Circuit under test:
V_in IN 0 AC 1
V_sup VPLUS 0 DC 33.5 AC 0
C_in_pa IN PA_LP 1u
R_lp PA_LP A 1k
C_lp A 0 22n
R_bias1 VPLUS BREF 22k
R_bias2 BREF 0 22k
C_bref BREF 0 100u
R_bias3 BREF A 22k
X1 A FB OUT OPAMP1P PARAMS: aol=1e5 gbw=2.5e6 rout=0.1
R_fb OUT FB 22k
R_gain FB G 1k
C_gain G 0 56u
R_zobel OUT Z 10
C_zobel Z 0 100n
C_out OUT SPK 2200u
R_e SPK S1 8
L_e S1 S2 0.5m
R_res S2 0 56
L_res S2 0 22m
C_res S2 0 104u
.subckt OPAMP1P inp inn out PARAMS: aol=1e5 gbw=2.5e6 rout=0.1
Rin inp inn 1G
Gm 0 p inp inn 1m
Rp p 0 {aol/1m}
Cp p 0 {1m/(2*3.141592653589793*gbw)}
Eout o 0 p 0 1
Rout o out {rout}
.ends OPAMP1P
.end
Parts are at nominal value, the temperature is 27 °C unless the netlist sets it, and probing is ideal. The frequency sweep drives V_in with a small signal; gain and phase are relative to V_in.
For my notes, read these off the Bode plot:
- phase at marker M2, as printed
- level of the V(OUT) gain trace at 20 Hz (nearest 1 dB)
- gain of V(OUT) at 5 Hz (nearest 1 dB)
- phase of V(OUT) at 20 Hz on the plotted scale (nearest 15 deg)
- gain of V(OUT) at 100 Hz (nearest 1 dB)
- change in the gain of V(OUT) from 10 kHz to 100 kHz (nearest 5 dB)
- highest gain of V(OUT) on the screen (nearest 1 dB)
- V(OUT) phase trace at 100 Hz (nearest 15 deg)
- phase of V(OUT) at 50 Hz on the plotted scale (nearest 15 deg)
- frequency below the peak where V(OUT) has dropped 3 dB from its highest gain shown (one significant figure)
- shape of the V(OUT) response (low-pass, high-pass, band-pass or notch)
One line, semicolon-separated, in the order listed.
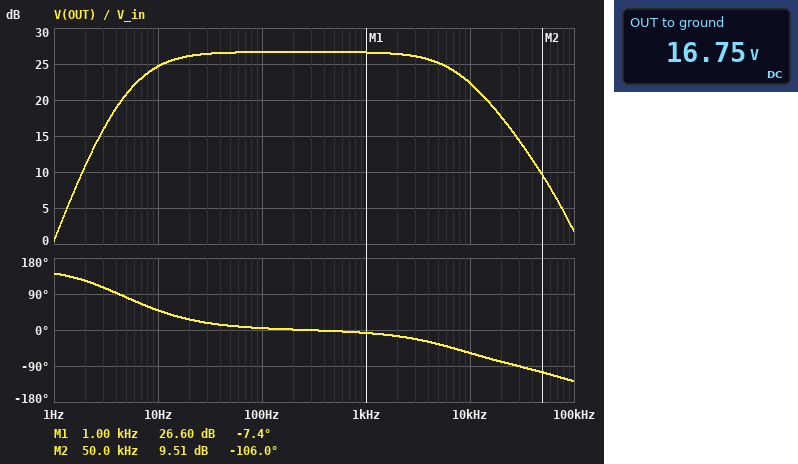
-106.0 deg; 26 dB; 21 dB; 30 deg; 27 dB; -20 dB; 27 dB; 0 deg; 15 deg; 8 Hz; band-pass
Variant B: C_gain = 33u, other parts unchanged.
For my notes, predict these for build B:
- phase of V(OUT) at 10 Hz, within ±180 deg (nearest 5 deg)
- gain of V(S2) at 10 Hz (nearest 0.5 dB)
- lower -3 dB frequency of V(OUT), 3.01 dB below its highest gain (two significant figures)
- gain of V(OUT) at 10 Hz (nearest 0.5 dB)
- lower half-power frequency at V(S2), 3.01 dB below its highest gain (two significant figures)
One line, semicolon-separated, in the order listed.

60 deg; 7.0 dB; 9.1 Hz; 24.0 dB; 39 Hz
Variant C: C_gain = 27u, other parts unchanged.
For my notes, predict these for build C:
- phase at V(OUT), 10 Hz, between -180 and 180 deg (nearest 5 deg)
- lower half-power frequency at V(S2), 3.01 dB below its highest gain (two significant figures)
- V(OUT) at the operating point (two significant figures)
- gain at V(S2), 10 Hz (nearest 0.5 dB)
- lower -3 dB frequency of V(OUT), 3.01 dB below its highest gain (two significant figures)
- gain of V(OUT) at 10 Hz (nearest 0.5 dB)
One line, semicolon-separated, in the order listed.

65 deg; 39 Hz; 17 V; 6.5 dB; 9.9 Hz; 23.5 dB
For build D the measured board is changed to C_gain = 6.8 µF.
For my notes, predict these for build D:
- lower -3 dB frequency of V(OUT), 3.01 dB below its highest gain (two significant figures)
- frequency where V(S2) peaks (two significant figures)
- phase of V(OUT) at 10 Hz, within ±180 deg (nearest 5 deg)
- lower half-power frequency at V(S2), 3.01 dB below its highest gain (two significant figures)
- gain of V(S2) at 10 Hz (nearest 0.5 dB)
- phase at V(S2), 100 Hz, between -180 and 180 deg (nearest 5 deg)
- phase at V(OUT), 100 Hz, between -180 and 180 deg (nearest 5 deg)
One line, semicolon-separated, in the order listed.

25 Hz; 110 Hz; 95 deg; 44 Hz; 0 dB; 20 deg; 15 deg
